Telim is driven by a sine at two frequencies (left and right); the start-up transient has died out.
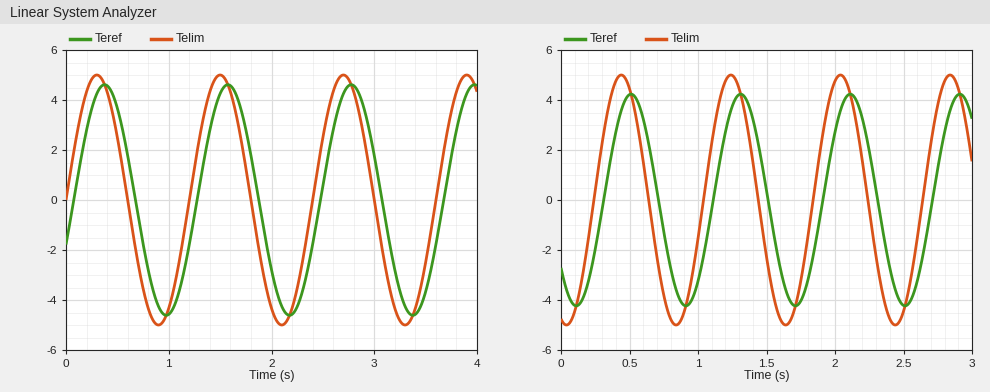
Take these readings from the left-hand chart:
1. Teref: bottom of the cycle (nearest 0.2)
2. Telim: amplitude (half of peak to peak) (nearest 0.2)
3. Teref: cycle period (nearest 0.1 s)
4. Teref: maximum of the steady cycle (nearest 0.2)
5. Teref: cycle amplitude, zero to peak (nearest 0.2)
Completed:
-4.6
5.0
1.2 s
4.6
4.6
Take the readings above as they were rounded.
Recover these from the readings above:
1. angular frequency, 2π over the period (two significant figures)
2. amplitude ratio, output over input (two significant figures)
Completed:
5.2 rad/s
0.92
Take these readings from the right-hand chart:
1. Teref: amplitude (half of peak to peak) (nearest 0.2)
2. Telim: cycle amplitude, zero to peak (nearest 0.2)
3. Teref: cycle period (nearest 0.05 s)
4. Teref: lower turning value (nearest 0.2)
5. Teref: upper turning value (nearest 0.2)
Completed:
4.2
5.0
0.80 s
-4.2
4.2
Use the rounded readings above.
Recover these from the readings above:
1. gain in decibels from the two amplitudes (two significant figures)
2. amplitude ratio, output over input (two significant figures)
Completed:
-1.5 dB
0.84
